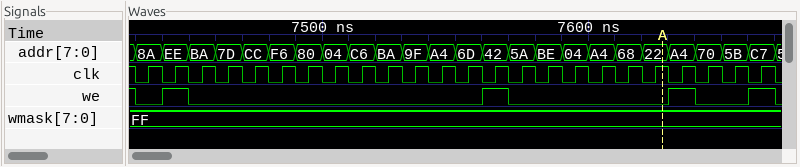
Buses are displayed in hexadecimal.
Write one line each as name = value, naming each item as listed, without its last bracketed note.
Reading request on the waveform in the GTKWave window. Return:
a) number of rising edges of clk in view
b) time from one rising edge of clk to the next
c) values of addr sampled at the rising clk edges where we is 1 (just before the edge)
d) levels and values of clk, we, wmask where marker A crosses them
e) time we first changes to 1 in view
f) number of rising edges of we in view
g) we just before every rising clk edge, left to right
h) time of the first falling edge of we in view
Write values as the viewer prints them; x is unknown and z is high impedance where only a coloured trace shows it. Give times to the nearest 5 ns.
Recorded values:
number of rising edges of clk in view = 24
time from one rising edge of clk to the next = 10 ns
values of addr sampled at the rising clk edges where we is 1 = EE, 42, A4, C7
levels and values of clk, we, wmask where marker A crosses them = clk=1, we=0, wmask=FF
time we first changes to 1 in view = 7440 ns
number of rising edges of we in view = 4
we just before every rising clk edge, left to right = 0 1 0 0 0 0 0 0 0 0 0 0 0 1 0 0 0 0 0 0 1 0 0 1
time of the first falling edge of we in view = 7430 ns
